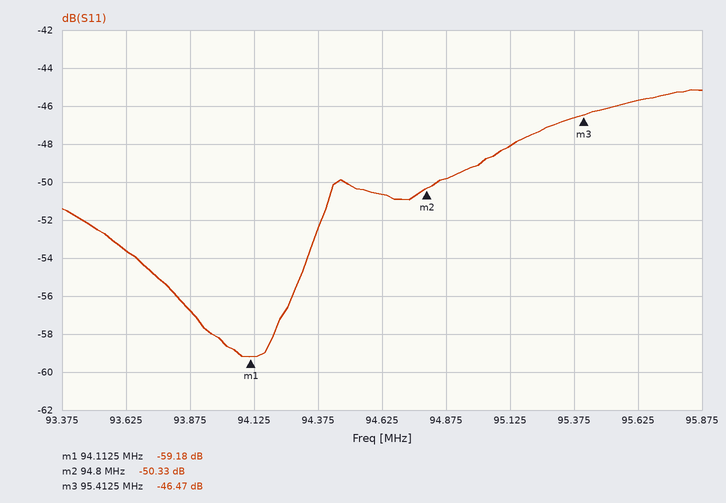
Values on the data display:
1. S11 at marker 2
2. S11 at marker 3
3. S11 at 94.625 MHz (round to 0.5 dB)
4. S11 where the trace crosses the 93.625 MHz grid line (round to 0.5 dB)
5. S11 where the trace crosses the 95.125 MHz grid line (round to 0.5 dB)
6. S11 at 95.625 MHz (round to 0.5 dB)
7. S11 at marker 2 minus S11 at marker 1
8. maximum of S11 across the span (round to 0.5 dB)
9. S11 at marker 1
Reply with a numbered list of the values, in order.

1. -50.33 dB
2. -46.47 dB
3. -50.5 dB
4. -53.5 dB
5. -48.0 dB
6. -45.5 dB
7. 8.85 dB
8. -45.0 dB
9. -59.18 dB
